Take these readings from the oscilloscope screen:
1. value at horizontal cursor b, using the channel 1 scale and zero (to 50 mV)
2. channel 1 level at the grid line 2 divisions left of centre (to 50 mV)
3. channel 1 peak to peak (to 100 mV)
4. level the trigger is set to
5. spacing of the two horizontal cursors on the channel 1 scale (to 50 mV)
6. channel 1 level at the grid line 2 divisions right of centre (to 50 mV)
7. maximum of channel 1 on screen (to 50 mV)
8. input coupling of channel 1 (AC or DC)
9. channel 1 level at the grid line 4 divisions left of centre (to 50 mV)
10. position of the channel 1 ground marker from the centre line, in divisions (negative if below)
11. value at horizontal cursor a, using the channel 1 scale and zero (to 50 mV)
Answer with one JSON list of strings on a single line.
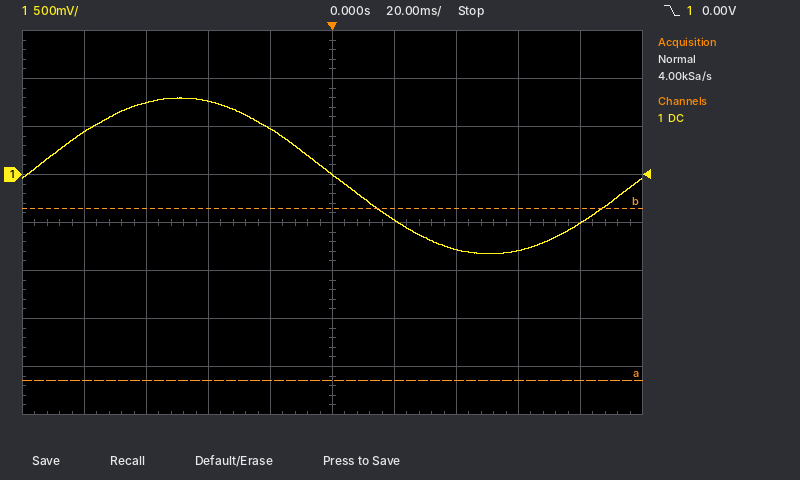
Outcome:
["-350 mV", "750 mV", "1.60 V", "0.00 V", "1.80 V", "-800 mV", "800 mV", "DC", "450 mV", "+1.0 div", "-2.15 V"]
